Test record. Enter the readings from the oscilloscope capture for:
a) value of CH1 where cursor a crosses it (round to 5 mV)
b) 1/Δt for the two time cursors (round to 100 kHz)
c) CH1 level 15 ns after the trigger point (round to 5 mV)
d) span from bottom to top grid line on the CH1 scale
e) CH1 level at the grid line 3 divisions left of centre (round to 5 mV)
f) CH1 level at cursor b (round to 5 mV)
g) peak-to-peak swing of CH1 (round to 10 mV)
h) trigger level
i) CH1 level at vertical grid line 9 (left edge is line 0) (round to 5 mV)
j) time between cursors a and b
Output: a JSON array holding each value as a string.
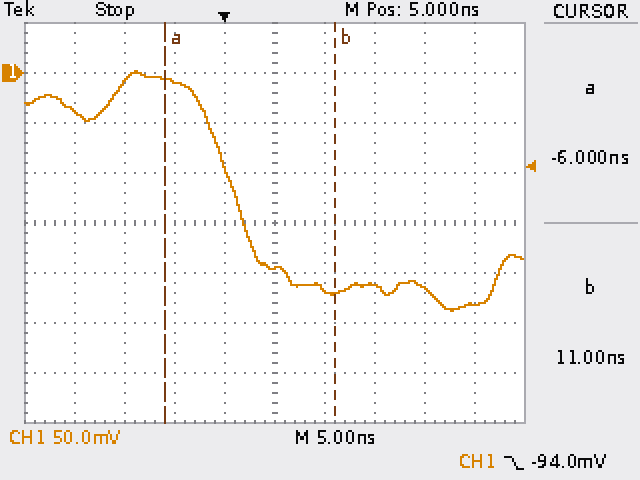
["-5 mV", "58.8 MHz", "-210 mV", "400 mV", "-10 mV", "-220 mV", "240 mV", "-94.0 mV", "-230 mV", "17.0 ns"]
